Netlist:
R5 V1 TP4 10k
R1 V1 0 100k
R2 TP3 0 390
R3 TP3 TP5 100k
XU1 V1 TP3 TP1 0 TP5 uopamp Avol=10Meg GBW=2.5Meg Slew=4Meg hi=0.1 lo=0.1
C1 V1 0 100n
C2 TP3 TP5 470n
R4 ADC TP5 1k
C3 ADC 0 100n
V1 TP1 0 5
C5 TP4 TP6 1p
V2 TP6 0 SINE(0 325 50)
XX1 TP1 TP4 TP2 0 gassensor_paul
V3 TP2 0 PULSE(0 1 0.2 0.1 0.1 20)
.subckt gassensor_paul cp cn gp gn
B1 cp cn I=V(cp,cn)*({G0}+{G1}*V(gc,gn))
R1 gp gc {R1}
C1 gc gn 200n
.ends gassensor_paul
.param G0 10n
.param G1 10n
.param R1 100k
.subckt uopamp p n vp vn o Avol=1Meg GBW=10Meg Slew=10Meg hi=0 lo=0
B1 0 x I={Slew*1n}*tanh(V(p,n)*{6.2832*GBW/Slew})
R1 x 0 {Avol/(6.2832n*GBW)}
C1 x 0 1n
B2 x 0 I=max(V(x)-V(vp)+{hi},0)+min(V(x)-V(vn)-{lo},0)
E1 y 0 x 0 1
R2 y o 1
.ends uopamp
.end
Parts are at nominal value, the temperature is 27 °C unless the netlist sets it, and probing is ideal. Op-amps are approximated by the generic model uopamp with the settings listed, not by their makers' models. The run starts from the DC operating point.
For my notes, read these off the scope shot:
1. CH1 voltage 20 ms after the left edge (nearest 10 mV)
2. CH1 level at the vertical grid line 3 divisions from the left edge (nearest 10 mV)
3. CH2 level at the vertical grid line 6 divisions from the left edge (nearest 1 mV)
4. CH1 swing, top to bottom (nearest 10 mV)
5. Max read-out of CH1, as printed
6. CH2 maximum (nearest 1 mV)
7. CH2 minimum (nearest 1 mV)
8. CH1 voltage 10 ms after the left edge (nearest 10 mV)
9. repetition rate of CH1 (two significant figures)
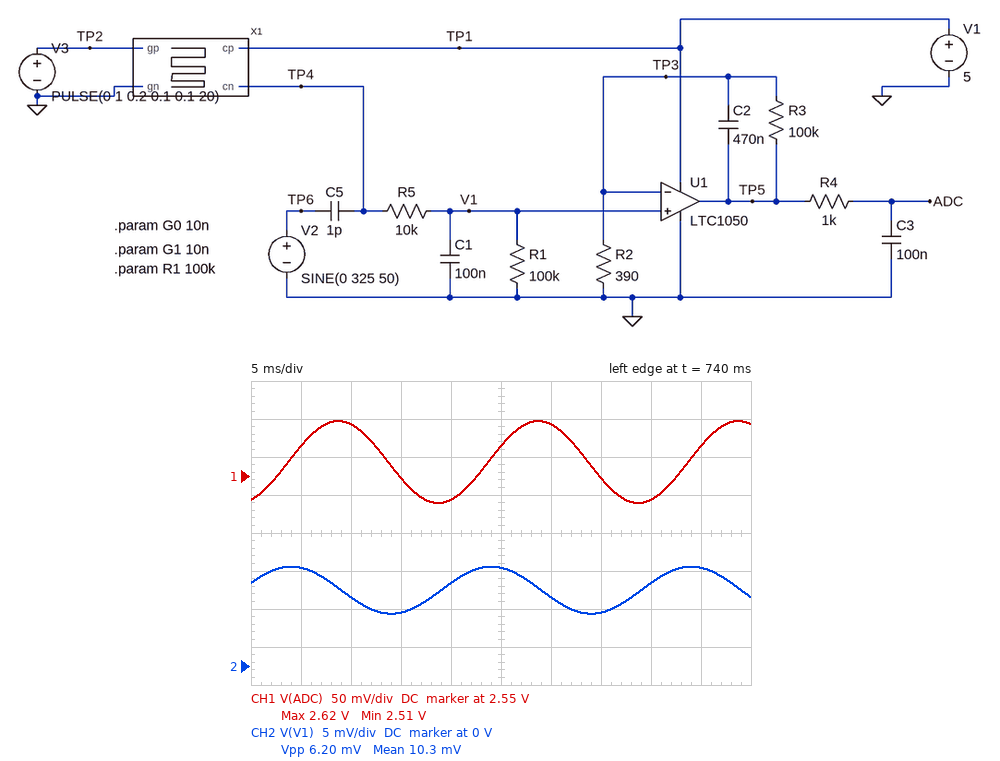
2.52 V
2.55 V
9 mV
110 mV
2.62 V
13 mV
7 mV
2.62 V
50 Hz
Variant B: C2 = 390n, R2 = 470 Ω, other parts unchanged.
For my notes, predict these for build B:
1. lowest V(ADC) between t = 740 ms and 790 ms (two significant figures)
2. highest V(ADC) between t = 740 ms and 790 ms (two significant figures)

2.1 V
2.2 V
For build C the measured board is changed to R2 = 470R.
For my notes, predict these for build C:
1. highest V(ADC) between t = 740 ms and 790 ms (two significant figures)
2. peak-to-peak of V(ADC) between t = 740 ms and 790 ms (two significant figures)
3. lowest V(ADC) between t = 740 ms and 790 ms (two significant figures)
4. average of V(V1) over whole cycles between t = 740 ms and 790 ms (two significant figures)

2.2 V
90 mV
2.1 V
10 mV
